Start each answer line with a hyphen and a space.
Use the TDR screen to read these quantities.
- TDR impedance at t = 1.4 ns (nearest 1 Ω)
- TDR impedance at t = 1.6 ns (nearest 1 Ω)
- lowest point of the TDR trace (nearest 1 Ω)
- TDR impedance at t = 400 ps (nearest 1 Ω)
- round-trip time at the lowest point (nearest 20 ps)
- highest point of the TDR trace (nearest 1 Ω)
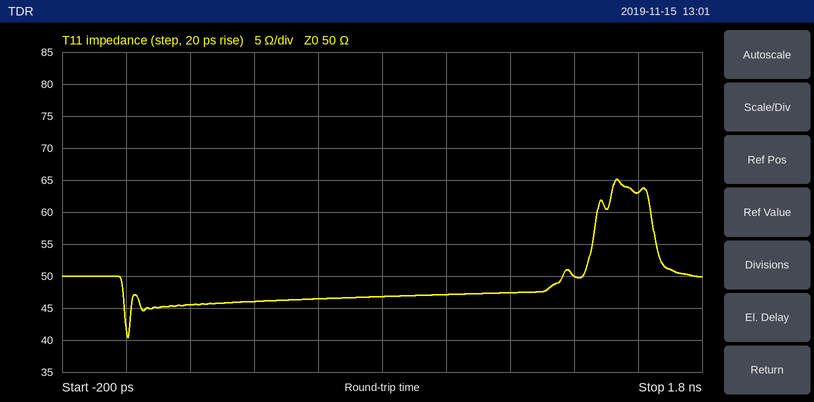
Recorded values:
- 50 Ω
- 63 Ω
- 40 Ω
- 46 Ω
- 0 ps
- 65 Ω
